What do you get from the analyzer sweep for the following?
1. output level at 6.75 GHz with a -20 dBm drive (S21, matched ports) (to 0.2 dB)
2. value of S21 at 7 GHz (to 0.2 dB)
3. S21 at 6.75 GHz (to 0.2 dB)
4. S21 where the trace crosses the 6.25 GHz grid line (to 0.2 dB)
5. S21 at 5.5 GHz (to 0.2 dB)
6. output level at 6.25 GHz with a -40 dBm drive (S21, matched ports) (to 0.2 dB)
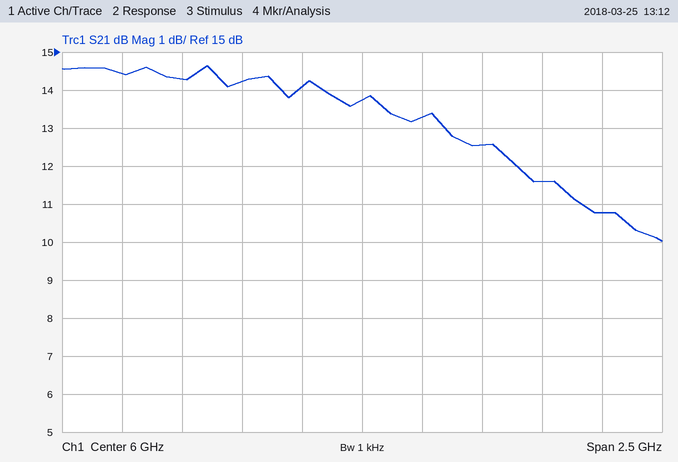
-8.4 dBm
10.8 dB
11.6 dB
13.2 dB
14.2 dB
-26.8 dBm
